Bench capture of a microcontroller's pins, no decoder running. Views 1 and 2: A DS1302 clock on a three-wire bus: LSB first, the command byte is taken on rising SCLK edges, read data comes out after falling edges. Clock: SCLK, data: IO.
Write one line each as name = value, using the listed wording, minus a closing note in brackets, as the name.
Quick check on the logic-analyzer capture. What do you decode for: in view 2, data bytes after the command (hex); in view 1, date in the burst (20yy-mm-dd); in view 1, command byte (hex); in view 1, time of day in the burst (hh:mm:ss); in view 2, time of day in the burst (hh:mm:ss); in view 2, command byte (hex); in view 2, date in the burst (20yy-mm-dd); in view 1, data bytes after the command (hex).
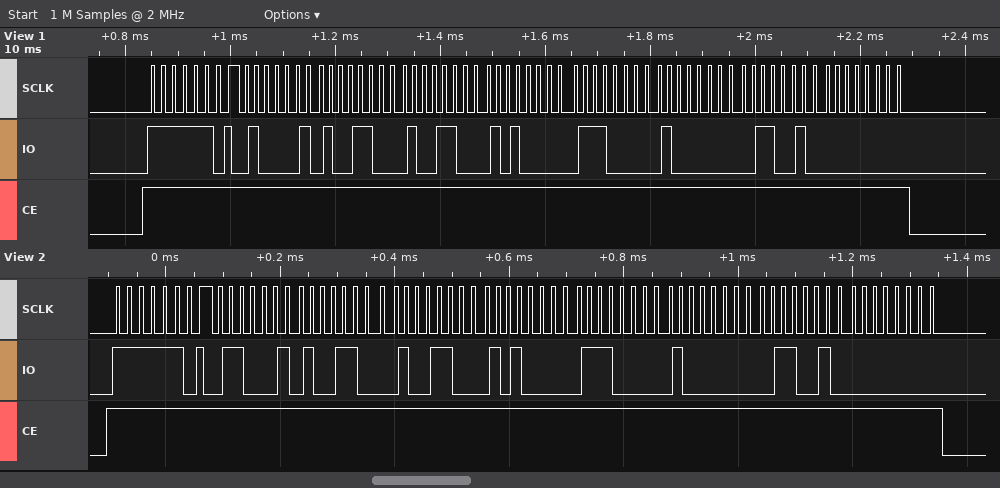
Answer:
in view 2, data bytes after the command = 46 19 19 05 07 01 26 00
in view 1, date in the burst = 2026-07-05
in view 1, command byte = 0xBF
in view 1, time of day in the burst = 19:19:42
in view 2, time of day in the burst = 19:19:46
in view 2, command byte = 0xBF
in view 2, date in the burst = 2026-07-05
in view 1, data bytes after the command = 42 19 19 05 07 01 26 00
